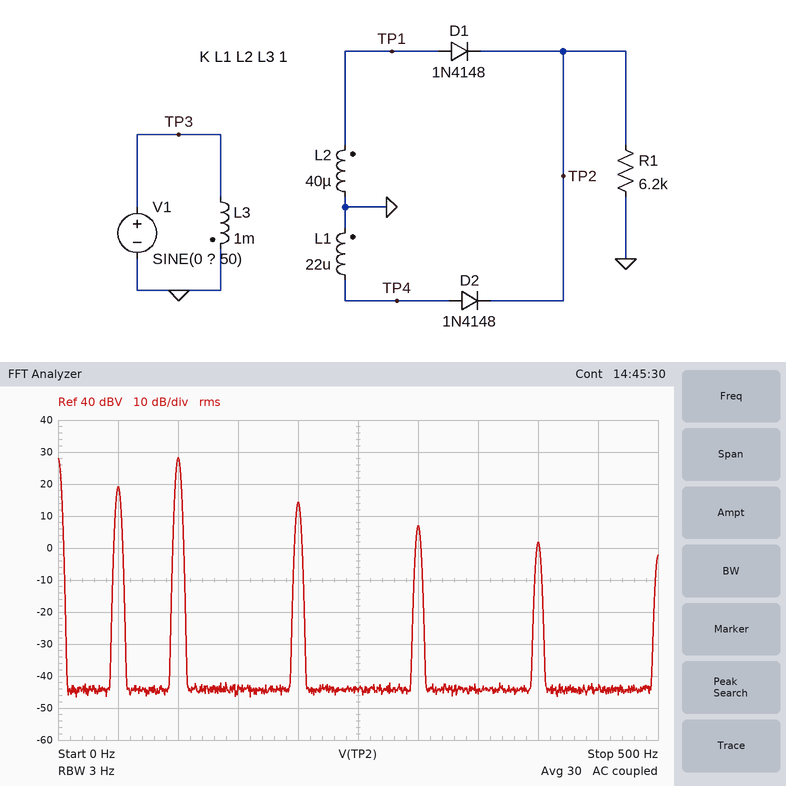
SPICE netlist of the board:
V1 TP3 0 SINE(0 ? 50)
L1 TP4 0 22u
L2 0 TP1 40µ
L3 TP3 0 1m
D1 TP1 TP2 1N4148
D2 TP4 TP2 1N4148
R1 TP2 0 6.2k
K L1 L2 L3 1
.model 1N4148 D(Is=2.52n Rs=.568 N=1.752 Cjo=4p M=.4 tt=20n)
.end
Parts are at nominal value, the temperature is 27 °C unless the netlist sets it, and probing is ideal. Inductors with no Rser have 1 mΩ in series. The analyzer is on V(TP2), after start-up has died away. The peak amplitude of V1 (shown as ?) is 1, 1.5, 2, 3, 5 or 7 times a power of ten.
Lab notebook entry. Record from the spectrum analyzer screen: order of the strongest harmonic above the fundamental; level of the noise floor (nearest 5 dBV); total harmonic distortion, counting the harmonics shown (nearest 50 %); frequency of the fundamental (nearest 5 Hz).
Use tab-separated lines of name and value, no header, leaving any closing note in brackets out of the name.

order of the strongest harmonic above the fundamental	2
level of the noise floor	-45 dBV
total harmonic distortion, counting the harmonics shown	300 %
frequency of the fundamental	50 Hz
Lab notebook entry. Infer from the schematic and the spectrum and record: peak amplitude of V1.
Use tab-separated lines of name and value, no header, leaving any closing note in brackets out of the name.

peak amplitude of V1	500 V
